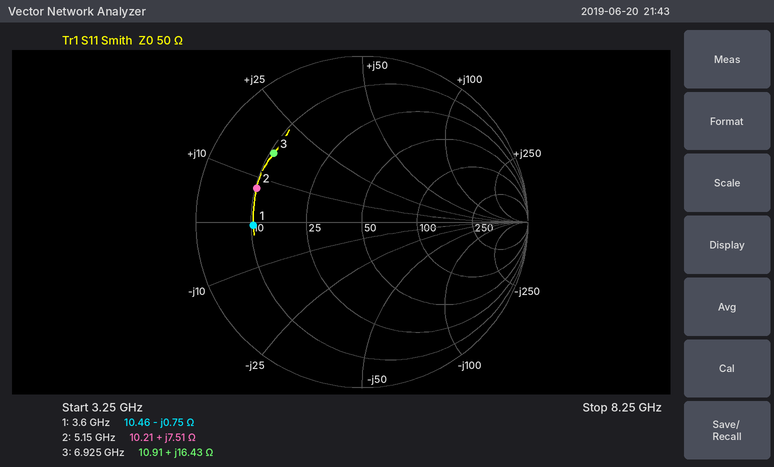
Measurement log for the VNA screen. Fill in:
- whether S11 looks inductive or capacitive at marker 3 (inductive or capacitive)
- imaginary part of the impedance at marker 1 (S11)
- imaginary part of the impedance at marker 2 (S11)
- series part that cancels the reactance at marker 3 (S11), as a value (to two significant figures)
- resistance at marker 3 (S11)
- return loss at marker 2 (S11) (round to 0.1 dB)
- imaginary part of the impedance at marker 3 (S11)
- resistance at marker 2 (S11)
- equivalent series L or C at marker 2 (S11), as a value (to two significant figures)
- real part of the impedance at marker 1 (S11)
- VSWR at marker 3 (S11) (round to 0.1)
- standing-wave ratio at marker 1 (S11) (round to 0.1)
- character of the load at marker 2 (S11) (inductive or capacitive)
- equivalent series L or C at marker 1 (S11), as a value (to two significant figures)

inductive
-0.75 Ω
+7.51 Ω
1.4 pF
10.91 Ω
3.5 dB
+16.43 Ω
10.21 Ω
230 pH
10.46 Ω
5.1
4.8
inductive
59 pF
